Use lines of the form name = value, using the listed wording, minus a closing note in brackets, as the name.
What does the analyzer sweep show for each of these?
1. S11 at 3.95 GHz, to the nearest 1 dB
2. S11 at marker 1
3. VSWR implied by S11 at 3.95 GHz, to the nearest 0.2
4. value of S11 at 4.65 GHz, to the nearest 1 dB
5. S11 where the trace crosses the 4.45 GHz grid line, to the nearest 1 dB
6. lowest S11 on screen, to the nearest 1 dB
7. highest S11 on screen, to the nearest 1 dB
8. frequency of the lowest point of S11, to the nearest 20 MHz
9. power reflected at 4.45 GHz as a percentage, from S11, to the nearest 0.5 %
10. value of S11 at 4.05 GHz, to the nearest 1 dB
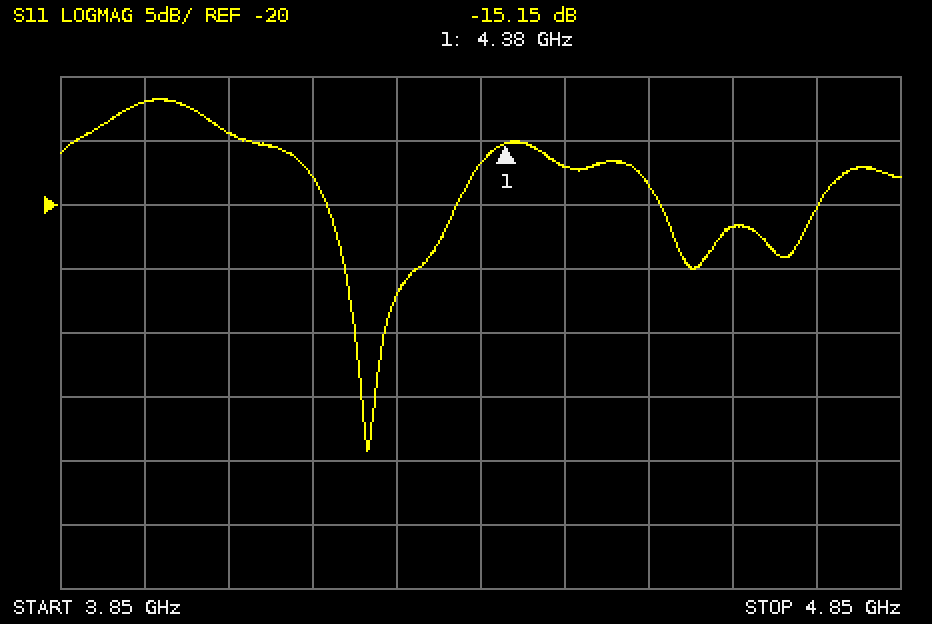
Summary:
S11 at 3.95 GHz, to the nearest 1 dB = -12 dB
S11 at marker 1 = -15.15 dB
VSWR implied by S11 at 3.95 GHz, to the nearest 0.2 = 1.6
value of S11 at 4.65 GHz, to the nearest 1 dB = -22 dB
S11 where the trace crosses the 4.45 GHz grid line, to the nearest 1 dB = -17 dB
lowest S11 on screen, to the nearest 1 dB = -39 dB
highest S11 on screen, to the nearest 1 dB = -12 dB
frequency of the lowest point of S11, to the nearest 20 MHz = 4.22 GHz
power reflected at 4.45 GHz as a percentage, from S11, to the nearest 0.5 % = 2.0 %
value of S11 at 4.05 GHz, to the nearest 1 dB = -14 dB
